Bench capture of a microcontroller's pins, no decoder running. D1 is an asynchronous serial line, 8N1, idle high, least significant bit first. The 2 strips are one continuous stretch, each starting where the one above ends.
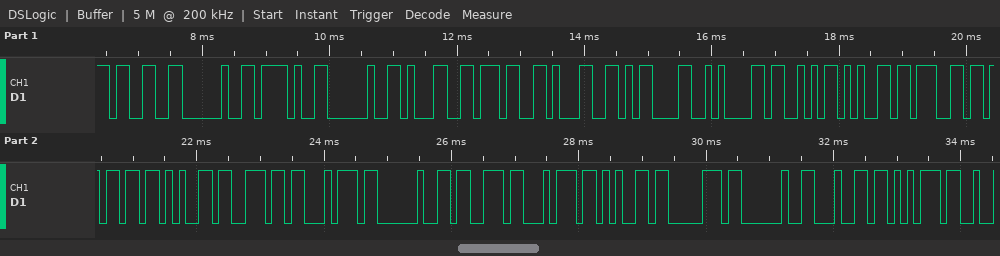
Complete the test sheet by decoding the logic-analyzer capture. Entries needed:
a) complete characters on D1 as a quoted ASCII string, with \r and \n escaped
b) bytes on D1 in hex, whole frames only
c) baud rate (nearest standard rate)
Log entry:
"3 / 171\r\nSegment step du"
33 20 2F 20 31 37 31 0D 0A 53 65 67 6D 65 6E 74 20 73 74 65 70 20 64 75
9600 baud
